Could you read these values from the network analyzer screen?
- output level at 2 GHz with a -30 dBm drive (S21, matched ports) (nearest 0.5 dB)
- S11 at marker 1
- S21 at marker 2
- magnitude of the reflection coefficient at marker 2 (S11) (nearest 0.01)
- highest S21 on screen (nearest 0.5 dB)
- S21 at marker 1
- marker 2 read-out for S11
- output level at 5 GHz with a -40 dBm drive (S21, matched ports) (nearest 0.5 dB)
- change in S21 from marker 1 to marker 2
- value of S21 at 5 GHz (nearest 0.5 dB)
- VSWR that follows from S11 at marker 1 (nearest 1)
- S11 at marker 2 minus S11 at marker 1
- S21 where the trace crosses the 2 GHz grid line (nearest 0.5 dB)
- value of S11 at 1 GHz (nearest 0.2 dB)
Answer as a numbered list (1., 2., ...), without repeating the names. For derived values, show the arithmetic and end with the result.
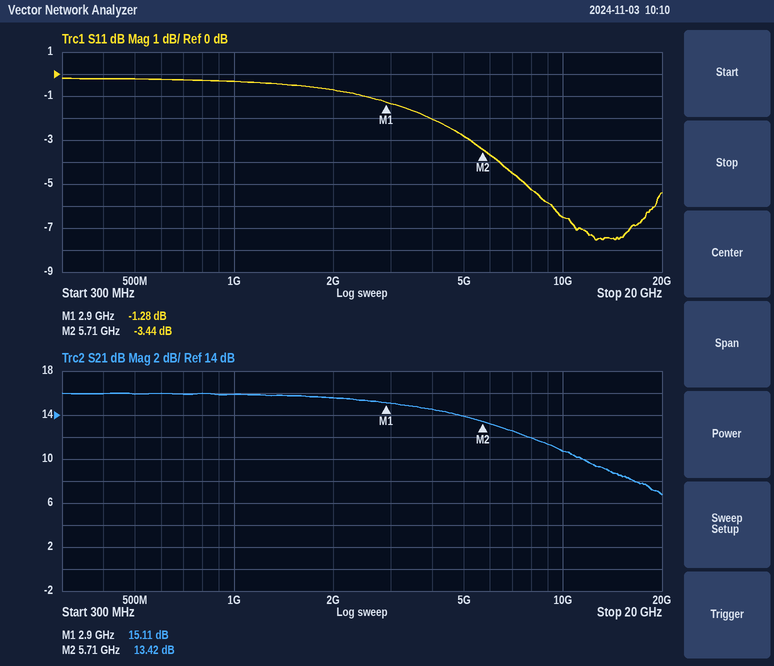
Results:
1. -30 dBm + (15.5 dB) = -14.5 dBm
2. -1.28 dB
3. 13.42 dB
4. 10^(-3.44/20) ≈ 0.67
5. 16.0 dB
6. 15.11 dB
7. -3.44 dB
8. -40 dBm + (14.0 dB) = -26.0 dBm
9. 13.42 − (15.11) = -1.69 dB
10. 14.0 dB
11. (1 + 0.8630)/(1 − 0.8630) ≈ 14
12. -3.44 − (-1.28) = -2.16 dB
13. 15.5 dB
14. -0.4 dB
